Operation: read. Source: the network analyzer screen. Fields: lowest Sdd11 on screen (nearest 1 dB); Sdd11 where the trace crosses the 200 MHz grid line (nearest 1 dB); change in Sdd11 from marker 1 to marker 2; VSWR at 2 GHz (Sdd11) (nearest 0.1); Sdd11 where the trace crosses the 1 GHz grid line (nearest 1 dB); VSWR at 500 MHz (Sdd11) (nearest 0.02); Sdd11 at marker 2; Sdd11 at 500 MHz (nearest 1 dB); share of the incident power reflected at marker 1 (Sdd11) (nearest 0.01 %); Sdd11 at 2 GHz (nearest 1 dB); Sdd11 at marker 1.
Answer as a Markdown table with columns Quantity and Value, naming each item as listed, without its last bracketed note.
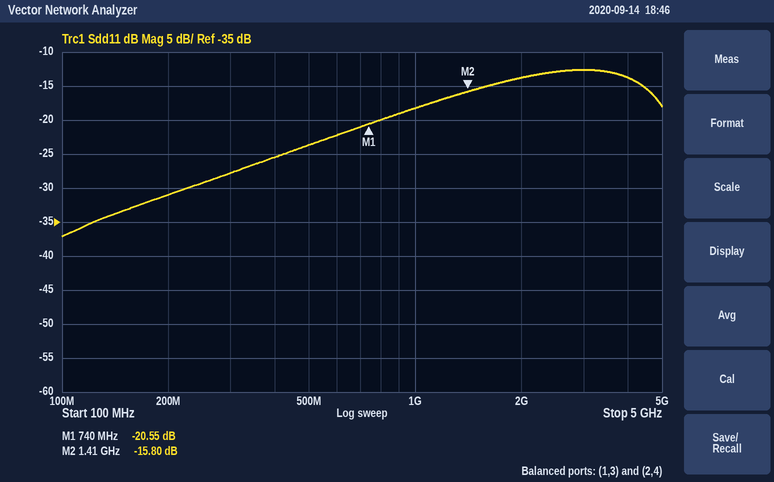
| Quantity | Value |
|---|---|
| lowest Sdd11 on screen | -37 dB |
| Sdd11 where the trace crosses the 200 MHz grid line | -31 dB |
| change in Sdd11 from marker 1 to marker 2 | 4.75 dB |
| VSWR at 2 GHz (Sdd11) | 1.5 |
| Sdd11 where the trace crosses the 1 GHz grid line | -18 dB |
| VSWR at 500 MHz (Sdd11) | 1.14 |
| Sdd11 at marker 2 | -15.80 dB |
| Sdd11 at 500 MHz | -24 dB |
| share of the incident power reflected at marker 1 (Sdd11) | 0.88 % |
| Sdd11 at 2 GHz | -14 dB |
| Sdd11 at marker 1 | -20.55 dB |
